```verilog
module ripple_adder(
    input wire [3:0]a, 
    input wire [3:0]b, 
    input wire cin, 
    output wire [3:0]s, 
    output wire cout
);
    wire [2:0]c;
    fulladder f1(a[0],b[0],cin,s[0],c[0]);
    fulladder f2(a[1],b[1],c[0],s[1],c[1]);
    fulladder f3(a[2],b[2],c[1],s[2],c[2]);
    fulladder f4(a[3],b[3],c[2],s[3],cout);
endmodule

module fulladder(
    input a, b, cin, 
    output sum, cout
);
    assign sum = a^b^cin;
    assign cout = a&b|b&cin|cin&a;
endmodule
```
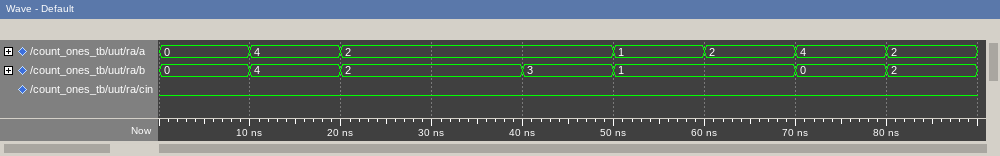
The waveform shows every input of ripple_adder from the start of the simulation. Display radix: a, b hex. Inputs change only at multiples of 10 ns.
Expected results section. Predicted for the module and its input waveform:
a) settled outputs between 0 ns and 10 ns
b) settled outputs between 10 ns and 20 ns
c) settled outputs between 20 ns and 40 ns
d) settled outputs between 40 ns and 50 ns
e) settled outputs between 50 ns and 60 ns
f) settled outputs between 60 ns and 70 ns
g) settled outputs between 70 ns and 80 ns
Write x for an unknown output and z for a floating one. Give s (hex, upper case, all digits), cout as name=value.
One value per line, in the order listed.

s=0, cout=0
s=8, cout=0
s=4, cout=0
s=5, cout=0
s=2, cout=0
s=3, cout=0
s=4, cout=0
